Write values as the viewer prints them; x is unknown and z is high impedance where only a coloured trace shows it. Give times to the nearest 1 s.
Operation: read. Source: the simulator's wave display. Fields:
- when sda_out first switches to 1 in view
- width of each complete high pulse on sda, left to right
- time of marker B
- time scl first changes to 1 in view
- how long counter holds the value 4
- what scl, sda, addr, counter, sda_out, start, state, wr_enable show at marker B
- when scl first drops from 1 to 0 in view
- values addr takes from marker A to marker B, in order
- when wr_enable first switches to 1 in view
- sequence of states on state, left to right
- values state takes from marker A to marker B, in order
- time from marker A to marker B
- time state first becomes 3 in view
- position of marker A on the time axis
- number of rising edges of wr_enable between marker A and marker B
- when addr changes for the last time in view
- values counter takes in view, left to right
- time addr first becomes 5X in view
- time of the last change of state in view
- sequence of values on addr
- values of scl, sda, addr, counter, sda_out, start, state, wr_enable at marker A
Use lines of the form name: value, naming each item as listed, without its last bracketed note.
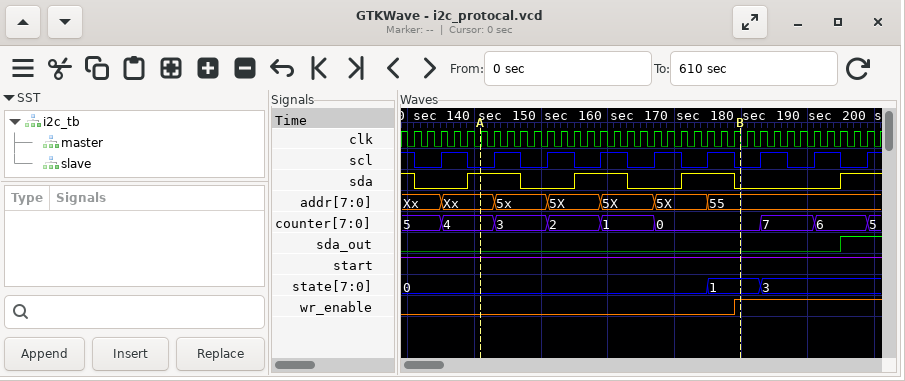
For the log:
when sda_out first switches to 1 in view: 195 s
width of each complete high pulse on sda, left to right: 8 s, 8 s, 8 s
time of marker B: 180 s
time scl first changes to 1 in view: 135 s
how long counter holds the value 4: 8 s
what scl, sda, addr, counter, sda_out, start, state, wr_enable show at marker B: scl=0, sda=0, addr=55, counter=0, sda_out=0, start=1, state=1, wr_enable=1
when scl first drops from 1 to 0 in view: 131 s
values addr takes from marker A to marker B, in order: Xx, 5x, 5X, 5X, 5X, 55
when wr_enable first switches to 1 in view: 179 s
sequence of states on state, left to right: 0, 1, 3
values state takes from marker A to marker B, in order: 0, 1
time from marker A to marker B: 39 s
time state first becomes 3 in view: 183 s
position of marker A on the time axis: 141 s
number of rising edges of wr_enable between marker A and marker B: 1
when addr changes for the last time in view: 175 s
values counter takes in view, left to right: 5, 4, 3, 2, 1, 0, 7, 6, 5
time addr first becomes 5X in view: 151 s
time of the last change of state in view: 183 s
sequence of values on addr: Xx, Xx, 5x, 5X, 5X, 5X, 55
values of scl, sda, addr, counter, sda_out, start, state, wr_enable at marker A: scl=0, sda=1, addr=Xx, counter=4, sda_out=0, start=1, state=0, wr_enable=0
